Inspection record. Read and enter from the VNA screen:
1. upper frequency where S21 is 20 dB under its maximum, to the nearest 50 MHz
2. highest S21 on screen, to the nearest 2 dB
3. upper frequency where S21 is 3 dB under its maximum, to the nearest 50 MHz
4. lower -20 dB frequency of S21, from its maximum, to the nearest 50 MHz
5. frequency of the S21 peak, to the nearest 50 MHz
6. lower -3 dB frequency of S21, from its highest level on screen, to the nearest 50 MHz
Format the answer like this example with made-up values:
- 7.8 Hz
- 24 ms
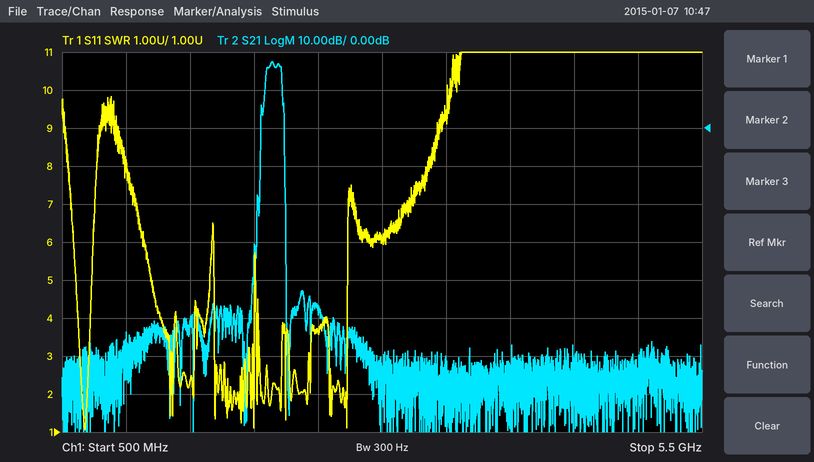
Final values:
- 2.25 GHz
- 18 dB
- 2.20 GHz
- 2.05 GHz
- 2.15 GHz
- 2.10 GHz
